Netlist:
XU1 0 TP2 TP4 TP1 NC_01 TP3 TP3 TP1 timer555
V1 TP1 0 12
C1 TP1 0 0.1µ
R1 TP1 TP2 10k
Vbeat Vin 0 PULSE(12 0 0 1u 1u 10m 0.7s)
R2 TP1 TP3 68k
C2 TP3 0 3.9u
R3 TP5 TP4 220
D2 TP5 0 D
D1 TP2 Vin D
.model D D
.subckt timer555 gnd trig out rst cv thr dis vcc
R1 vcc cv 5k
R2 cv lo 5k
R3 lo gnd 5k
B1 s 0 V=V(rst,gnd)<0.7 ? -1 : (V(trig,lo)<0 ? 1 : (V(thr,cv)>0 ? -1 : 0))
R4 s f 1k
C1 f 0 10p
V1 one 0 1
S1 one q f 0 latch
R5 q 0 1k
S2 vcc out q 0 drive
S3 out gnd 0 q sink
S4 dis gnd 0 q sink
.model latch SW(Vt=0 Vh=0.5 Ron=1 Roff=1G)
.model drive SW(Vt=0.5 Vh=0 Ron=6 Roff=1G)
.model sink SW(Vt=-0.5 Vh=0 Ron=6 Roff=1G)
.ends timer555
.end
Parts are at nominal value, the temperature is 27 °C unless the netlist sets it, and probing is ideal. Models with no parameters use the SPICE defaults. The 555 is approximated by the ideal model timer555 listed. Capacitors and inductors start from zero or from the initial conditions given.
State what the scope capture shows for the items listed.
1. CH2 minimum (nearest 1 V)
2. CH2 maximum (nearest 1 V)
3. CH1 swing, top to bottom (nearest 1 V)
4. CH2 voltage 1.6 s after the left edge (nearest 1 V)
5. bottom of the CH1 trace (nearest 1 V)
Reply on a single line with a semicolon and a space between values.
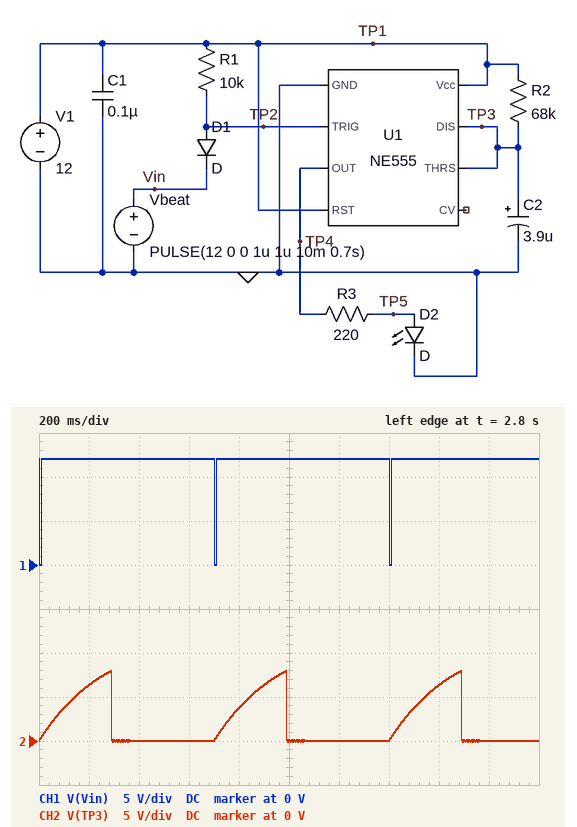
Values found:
0 V; 8 V; 12 V; 6 V; 0 V
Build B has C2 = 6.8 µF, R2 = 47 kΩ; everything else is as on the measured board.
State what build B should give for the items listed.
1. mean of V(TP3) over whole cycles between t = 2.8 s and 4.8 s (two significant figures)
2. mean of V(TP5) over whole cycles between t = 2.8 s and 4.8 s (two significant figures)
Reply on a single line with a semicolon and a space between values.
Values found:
2.4 V; 380 mV
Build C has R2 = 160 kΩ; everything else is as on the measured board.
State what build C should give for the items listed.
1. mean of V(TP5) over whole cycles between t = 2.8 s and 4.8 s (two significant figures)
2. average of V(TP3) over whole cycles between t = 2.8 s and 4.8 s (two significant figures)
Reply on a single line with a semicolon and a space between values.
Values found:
740 mV; 4.6 V
